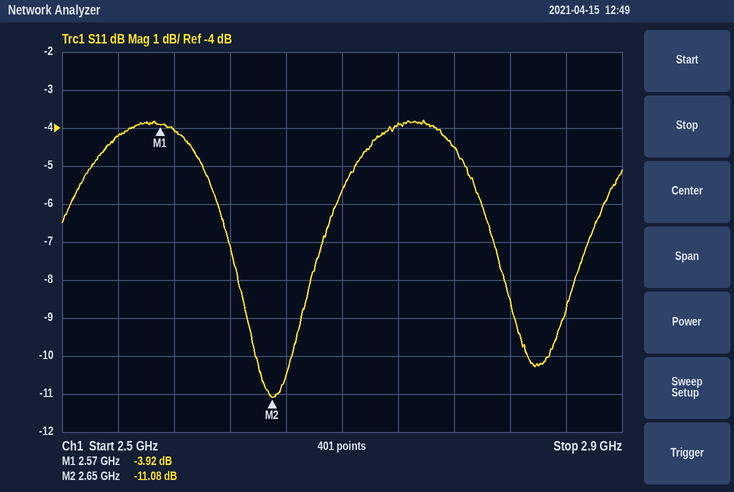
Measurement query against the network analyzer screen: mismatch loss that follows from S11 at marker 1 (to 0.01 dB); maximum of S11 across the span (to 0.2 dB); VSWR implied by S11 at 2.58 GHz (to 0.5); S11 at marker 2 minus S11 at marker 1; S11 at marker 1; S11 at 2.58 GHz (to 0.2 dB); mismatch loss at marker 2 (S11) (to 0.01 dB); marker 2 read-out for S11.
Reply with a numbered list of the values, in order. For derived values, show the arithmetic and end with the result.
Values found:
1. −10 log10(1 − 10^(-3.92/10)) ≈ 2.26 dB
2. -3.8 dB
3. |Γ| = 10^(-4/20) = 0.6310; VSWR = (1 + 0.6310)/(1 − 0.6310) ≈ 4.42, so 4.5 to the nearest 0.5
4. -11.08 − (-3.92) = -7.16 dB
5. -3.92 dB
6. -4.0 dB
7. −10 log10(1 − 10^(-11.08/10)) ≈ 0.35 dB
8. -11.08 dB
